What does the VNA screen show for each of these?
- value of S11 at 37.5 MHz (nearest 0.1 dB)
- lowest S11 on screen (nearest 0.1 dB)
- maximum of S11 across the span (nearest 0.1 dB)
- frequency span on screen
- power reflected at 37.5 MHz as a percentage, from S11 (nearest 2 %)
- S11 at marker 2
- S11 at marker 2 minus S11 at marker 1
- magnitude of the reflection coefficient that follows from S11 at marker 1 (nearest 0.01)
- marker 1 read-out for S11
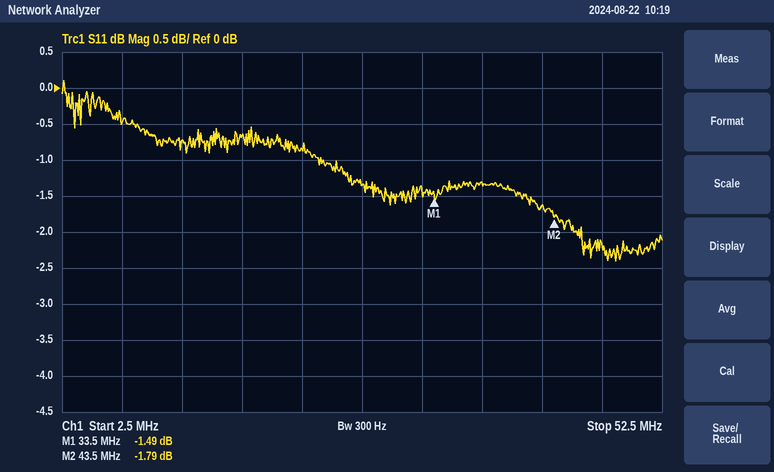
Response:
-1.3 dB
-2.4 dB
0.1 dB
50 MHz
74 %
-1.79 dB
-0.30 dB
0.84
-1.49 dB
